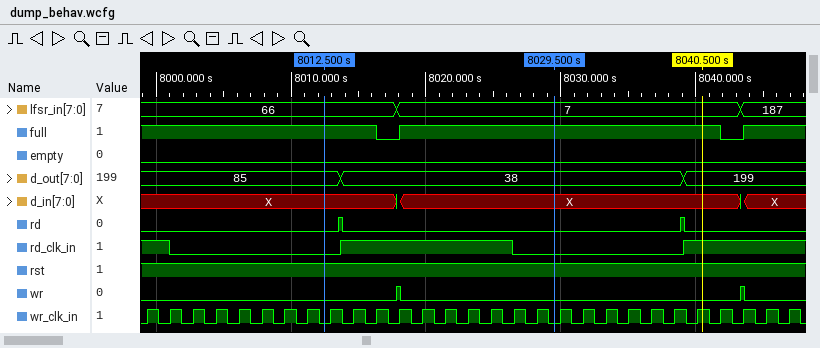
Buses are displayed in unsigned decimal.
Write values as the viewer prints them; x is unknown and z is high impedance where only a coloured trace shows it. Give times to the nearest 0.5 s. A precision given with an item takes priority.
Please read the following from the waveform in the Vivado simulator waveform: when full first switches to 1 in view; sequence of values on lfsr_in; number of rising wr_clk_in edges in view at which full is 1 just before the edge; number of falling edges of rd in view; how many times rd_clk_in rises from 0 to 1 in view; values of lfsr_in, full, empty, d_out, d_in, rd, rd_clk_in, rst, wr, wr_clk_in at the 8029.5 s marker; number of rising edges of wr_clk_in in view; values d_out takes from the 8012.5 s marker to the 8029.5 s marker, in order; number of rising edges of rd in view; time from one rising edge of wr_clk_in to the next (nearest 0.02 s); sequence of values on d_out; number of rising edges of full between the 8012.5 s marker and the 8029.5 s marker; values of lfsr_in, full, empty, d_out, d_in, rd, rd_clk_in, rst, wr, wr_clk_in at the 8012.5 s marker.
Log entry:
8018 s
66, 7, 187
27
2
2
lfsr_in=7, full=1, empty=0, d_out=38, d_in=X, rd=0, rd_clk_in=0, rst=1, wr=0, wr_clk_in=0
29
85, 38
2
1.7 s
85, 38, 199
1
lfsr_in=66, full=1, empty=0, d_out=85, d_in=X, rd=0, rd_clk_in=0, rst=1, wr=0, wr_clk_in=0
